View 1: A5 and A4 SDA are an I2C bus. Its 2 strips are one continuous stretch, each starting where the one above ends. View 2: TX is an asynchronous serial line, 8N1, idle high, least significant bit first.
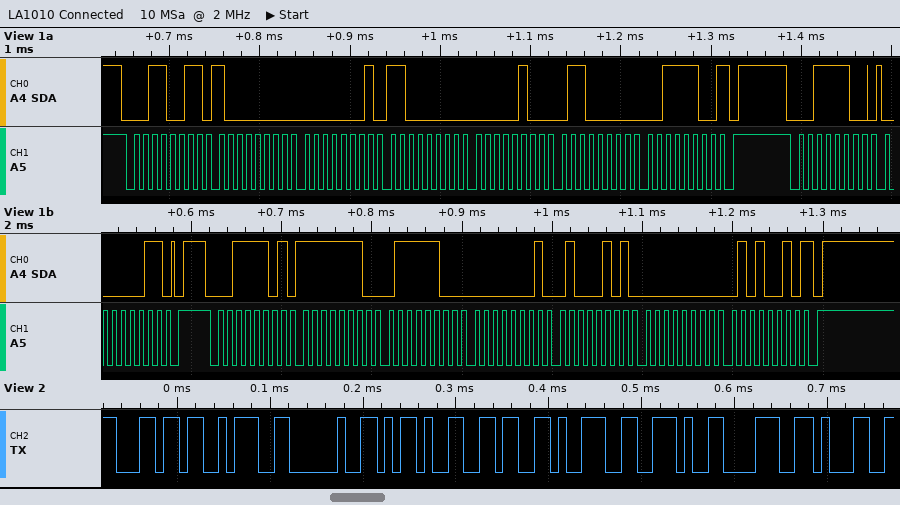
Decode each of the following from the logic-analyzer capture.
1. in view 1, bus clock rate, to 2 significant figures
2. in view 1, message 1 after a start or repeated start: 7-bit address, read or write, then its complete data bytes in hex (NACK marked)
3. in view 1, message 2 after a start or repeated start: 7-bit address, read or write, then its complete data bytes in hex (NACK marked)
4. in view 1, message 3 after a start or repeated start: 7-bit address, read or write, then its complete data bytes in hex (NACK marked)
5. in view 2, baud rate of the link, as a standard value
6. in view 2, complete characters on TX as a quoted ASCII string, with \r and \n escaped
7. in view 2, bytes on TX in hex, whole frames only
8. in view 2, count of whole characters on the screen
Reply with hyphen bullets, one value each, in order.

- 100 kHz
- 0x19 read: 80 01 C0 04 60 3C NACK
- 0x1E write: 03
- 0x1E read: FE 7C 01 45 00 52 NACK
- 115200 baud
- "l: -69.81"
- 0x6C 0x3A 0x20 0x2D 0x36 0x39 0x2E 0x38 0x31
- 9
